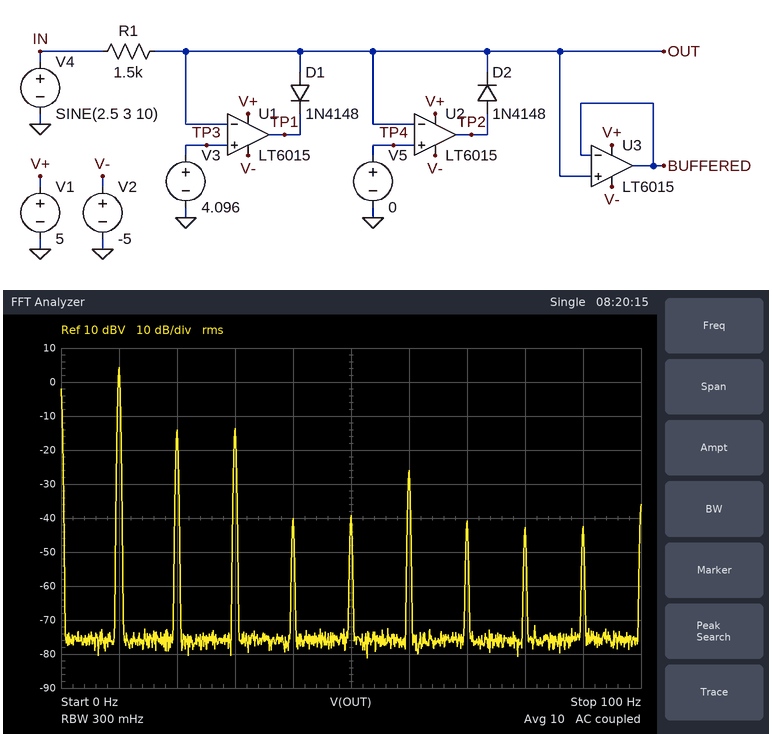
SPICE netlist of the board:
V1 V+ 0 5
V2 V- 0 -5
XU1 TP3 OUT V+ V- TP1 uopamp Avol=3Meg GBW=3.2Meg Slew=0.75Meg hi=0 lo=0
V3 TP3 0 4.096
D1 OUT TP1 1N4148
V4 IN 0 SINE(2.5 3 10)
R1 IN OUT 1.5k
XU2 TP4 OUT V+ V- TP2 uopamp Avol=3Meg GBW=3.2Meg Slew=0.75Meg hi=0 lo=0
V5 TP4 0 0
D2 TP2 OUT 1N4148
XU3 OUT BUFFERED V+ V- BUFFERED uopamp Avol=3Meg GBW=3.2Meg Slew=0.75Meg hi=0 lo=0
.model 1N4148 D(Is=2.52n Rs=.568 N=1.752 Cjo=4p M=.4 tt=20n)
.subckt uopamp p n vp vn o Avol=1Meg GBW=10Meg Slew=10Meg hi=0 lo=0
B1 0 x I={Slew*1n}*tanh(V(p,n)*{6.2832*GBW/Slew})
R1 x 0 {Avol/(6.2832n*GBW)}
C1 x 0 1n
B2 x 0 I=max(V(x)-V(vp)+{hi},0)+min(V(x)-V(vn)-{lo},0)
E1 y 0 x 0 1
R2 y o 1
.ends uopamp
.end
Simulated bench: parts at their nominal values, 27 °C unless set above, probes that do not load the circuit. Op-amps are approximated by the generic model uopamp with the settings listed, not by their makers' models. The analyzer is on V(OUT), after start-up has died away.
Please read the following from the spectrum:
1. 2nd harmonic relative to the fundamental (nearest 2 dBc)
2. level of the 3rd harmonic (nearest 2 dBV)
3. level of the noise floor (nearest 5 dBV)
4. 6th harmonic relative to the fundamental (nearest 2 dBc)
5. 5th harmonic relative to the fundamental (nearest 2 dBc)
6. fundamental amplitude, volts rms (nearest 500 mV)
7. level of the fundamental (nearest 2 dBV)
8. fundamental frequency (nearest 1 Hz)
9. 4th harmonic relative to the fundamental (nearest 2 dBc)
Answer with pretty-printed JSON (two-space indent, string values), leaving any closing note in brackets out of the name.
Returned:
{
  "2nd harmonic relative to the fundamental": "-18 dBc",
  "level of the 3rd harmonic": "-14 dBV",
  "level of the noise floor": "-75 dBV",
  "6th harmonic relative to the fundamental": "-30 dBc",
  "5th harmonic relative to the fundamental": "-44 dBc",
  "fundamental amplitude, volts rms": "1.5 V",
  "level of the fundamental": "4 dBV",
  "fundamental frequency": "10 Hz",
  "4th harmonic relative to the fundamental": "-44 dBc"
}
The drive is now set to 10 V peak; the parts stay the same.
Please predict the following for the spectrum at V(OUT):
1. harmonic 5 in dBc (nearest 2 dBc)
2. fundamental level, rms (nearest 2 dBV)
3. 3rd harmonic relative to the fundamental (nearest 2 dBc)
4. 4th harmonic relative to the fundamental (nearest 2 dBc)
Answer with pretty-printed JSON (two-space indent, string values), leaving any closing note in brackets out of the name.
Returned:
{
  "harmonic 5 in dBc": "-16 dBc",
  "fundamental level, rms": "6 dBV",
  "3rd harmonic relative to the fundamental": "-10 dBc",
  "4th harmonic relative to the fundamental": "-28 dBc"
}
